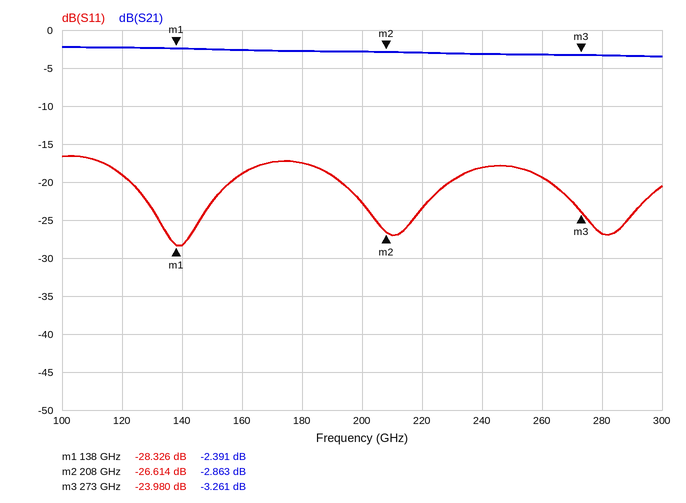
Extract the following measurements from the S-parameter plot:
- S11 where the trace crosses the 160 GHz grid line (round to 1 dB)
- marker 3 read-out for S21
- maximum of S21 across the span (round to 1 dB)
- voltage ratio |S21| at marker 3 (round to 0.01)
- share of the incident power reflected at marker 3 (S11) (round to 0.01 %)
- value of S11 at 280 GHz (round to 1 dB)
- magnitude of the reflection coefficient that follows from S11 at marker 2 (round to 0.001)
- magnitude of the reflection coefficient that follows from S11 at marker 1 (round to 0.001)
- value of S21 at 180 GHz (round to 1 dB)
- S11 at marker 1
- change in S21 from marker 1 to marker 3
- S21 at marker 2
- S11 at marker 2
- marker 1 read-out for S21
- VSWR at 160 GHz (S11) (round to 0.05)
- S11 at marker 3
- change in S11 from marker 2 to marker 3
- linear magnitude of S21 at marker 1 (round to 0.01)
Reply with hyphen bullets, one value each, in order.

- -19 dB
- -3.261 dB
- -2 dB
- 0.69
- 0.40 %
- -27 dB
- 0.047
- 0.038
- -3 dB
- -28.326 dB
- -0.870 dB
- -2.863 dB
- -26.614 dB
- -2.391 dB
- 1.25
- -23.980 dB
- 2.634 dB
- 0.76
